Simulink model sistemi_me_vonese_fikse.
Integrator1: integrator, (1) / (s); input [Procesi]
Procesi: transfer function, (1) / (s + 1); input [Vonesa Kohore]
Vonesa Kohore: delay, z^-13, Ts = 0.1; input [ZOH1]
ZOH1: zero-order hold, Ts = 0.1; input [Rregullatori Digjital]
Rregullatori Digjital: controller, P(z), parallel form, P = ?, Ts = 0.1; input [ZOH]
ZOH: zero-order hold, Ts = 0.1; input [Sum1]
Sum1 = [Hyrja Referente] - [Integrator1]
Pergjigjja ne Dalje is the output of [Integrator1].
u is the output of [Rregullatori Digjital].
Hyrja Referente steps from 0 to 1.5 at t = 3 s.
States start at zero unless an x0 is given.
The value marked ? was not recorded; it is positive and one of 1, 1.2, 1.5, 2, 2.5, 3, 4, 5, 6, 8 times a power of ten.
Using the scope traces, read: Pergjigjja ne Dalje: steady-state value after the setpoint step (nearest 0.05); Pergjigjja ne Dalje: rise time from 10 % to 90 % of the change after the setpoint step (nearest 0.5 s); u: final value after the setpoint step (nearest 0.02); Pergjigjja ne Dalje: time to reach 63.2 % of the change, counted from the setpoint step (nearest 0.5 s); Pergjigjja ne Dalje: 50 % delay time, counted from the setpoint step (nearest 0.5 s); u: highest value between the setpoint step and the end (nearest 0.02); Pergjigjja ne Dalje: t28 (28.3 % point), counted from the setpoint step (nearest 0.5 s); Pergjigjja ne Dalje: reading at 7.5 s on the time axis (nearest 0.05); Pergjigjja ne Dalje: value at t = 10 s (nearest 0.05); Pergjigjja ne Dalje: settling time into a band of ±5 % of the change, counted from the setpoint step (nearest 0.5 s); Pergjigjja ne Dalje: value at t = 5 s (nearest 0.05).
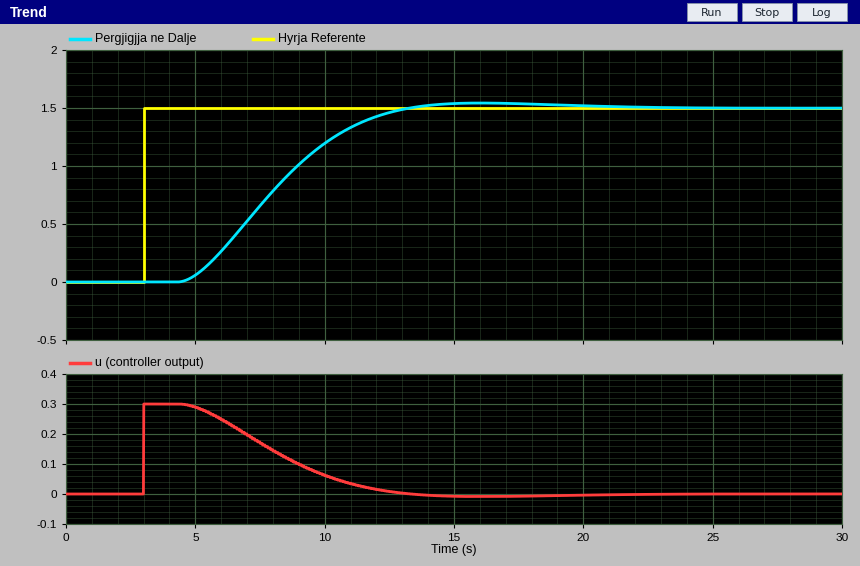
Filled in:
1.50
5.5 s
0.00
5.5 s
5.0 s
0.30
3.5 s
0.65
1.20
9.0 s
0.05
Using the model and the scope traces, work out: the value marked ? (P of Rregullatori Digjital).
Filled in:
0.2
